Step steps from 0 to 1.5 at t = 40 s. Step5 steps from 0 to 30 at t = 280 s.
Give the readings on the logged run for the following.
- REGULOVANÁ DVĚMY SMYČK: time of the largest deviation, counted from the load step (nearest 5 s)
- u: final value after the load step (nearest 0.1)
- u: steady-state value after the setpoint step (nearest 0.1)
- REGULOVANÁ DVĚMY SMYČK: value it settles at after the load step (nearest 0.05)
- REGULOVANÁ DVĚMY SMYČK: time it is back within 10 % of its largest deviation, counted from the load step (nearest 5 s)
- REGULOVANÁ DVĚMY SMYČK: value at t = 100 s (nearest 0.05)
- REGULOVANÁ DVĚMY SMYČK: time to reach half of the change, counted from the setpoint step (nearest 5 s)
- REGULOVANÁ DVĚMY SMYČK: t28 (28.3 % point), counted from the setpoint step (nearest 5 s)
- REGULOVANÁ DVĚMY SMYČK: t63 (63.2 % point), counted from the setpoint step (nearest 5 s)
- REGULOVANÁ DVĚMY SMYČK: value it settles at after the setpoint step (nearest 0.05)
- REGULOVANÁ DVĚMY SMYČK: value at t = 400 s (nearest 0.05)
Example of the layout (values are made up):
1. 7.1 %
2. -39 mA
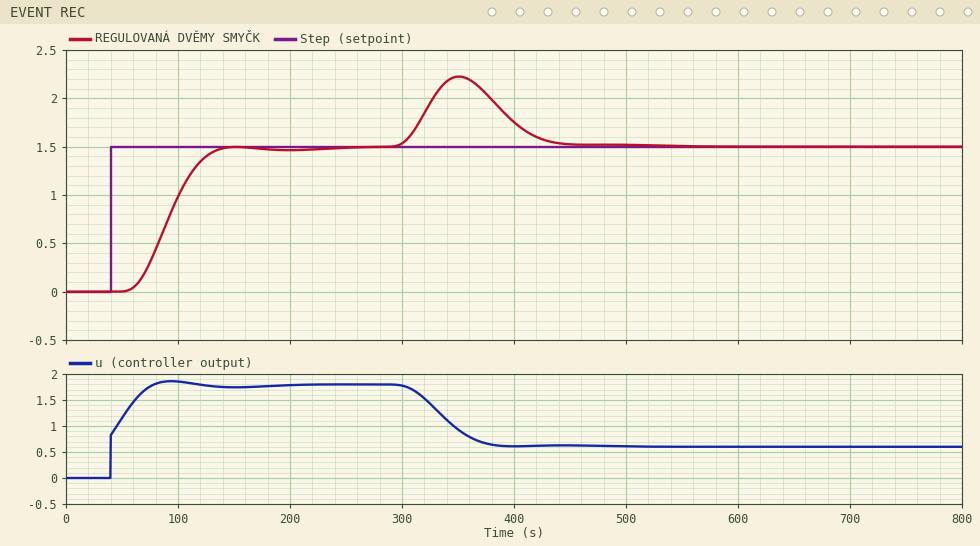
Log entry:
1. 70 s
2. 0.6
3. 1.8
4. 1.50
5. 145 s
6. 1.00
7. 50 s
8. 40 s
9. 60 s
10. 1.50
11. 1.75
